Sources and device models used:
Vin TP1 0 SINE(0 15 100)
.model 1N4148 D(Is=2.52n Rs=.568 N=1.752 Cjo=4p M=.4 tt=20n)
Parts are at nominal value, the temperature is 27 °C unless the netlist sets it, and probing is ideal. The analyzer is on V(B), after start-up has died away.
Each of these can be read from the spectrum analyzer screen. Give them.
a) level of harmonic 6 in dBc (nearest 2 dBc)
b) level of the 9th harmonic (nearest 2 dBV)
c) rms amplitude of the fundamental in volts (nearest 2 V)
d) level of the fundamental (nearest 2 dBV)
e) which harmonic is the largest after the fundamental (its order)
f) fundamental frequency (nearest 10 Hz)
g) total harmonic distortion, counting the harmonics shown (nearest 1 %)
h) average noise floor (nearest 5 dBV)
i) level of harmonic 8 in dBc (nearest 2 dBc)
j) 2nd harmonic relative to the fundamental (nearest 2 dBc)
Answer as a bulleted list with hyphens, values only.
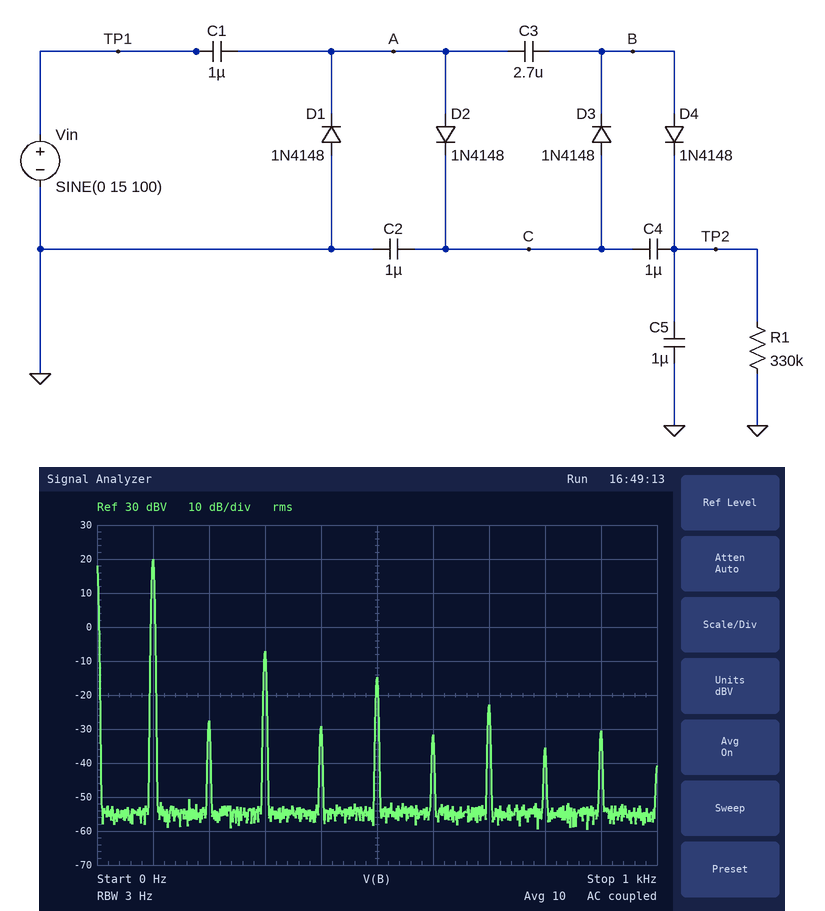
- -52 dBc
- -30 dBV
- 10 V
- 20 dBV
- 3
- 100 Hz
- 5 %
- -55 dBV
- -56 dBc
- -48 dBc
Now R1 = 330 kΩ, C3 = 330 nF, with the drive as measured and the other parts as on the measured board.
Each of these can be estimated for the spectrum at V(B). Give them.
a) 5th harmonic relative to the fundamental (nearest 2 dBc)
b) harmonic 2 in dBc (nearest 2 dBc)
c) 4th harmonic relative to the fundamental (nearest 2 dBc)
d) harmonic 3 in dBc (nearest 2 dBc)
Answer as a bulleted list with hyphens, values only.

- -32 dBc
- -44 dBc
- -48 dBc
- -22 dBc
